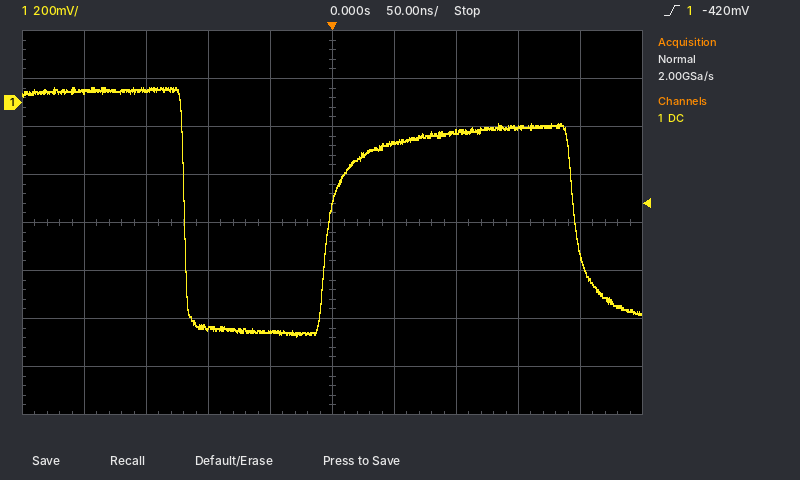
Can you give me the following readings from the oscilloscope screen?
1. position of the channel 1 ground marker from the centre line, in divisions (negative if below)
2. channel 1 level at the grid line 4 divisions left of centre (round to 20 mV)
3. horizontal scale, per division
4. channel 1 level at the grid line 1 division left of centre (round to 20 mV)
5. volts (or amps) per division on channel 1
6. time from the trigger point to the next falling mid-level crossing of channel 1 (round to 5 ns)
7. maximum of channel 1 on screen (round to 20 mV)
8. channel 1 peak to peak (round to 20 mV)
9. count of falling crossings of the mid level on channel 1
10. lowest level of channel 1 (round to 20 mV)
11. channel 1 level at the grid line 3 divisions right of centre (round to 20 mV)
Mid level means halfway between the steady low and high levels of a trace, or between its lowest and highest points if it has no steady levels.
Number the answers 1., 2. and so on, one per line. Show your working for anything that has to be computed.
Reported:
1. +2.5 div
2. 40 mV
3. 50 ns
4. -960 mV
5. 200 mV
6. 195 ns
7. 60 mV
8. 60 mV − (-980 mV) = 1.04 V
9. 2
10. -980 mV
11. -100 mV
